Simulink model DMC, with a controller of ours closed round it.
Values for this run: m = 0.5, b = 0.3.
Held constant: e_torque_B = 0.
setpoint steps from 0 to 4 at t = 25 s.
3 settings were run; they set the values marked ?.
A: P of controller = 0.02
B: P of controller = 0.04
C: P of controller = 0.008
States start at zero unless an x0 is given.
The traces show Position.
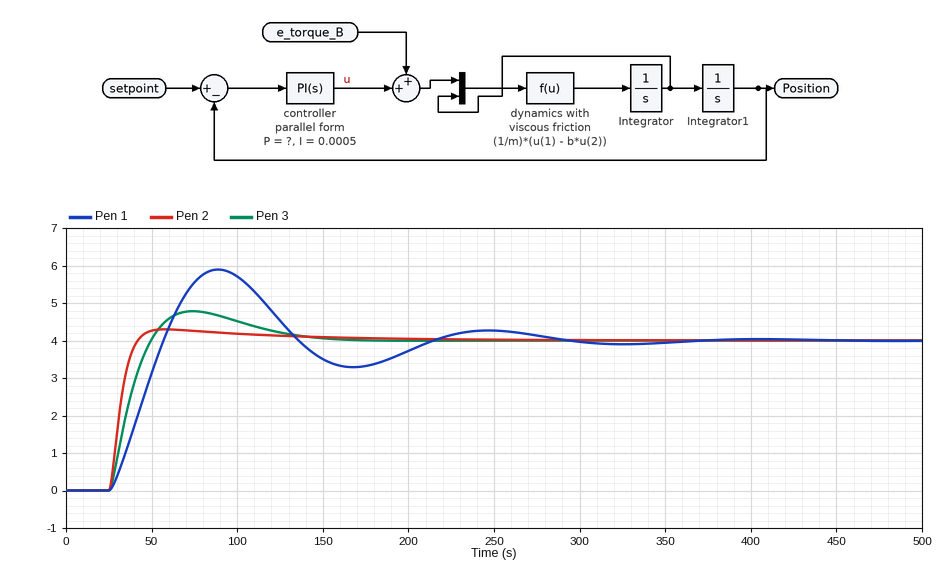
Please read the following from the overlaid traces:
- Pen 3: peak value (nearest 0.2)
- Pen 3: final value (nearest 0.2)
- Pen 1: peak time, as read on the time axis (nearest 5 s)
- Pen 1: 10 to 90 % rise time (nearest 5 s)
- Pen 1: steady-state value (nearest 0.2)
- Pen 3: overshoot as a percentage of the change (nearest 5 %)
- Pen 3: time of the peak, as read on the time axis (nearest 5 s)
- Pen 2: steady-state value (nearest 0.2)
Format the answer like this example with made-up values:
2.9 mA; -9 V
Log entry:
4.8; 4.0; 90 s; 25 s; 4.0; 20 %; 75 s; 4.0
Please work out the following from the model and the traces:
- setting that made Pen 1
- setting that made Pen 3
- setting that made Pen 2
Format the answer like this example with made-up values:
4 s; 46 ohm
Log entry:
C; A; B
